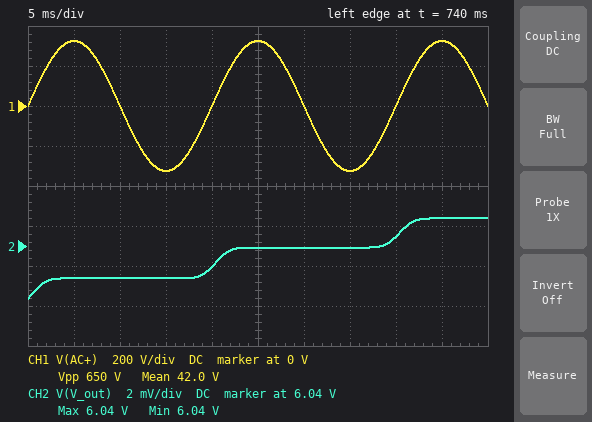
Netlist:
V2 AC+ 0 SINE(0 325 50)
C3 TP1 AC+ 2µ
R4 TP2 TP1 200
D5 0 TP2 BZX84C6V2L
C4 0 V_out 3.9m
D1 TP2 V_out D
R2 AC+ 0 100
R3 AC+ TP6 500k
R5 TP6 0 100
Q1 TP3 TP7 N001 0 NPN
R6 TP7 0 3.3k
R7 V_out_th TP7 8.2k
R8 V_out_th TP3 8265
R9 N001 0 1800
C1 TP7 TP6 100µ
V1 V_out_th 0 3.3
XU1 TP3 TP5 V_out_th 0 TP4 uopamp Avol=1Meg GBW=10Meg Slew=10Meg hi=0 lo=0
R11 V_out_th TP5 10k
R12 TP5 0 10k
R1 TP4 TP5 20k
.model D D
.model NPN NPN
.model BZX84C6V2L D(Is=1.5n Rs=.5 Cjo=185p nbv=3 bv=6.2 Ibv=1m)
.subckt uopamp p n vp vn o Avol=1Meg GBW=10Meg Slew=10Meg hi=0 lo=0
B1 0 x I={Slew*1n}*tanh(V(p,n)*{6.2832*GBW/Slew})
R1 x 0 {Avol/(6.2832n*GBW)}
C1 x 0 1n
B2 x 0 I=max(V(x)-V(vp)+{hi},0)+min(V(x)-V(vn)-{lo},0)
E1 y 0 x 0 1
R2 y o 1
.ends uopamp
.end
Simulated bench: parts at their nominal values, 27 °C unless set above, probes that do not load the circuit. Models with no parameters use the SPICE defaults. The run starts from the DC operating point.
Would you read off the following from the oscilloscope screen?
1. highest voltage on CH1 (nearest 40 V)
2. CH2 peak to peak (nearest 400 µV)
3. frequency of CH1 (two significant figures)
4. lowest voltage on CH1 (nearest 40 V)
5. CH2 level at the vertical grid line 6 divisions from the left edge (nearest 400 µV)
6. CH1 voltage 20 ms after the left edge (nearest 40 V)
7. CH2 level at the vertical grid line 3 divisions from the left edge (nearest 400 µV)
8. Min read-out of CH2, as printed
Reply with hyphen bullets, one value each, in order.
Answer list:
- 320 V
- 4.0 mV
- 50 Hz
- -320 V
- 6.0400 V
- 0 V
- 6.0384 V
- 6.04 V
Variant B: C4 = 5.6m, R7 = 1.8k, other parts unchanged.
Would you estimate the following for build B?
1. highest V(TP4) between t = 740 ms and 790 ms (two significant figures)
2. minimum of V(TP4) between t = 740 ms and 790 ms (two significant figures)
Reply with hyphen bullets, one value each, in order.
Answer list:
- -8.7 mV
- -9.6 mV
